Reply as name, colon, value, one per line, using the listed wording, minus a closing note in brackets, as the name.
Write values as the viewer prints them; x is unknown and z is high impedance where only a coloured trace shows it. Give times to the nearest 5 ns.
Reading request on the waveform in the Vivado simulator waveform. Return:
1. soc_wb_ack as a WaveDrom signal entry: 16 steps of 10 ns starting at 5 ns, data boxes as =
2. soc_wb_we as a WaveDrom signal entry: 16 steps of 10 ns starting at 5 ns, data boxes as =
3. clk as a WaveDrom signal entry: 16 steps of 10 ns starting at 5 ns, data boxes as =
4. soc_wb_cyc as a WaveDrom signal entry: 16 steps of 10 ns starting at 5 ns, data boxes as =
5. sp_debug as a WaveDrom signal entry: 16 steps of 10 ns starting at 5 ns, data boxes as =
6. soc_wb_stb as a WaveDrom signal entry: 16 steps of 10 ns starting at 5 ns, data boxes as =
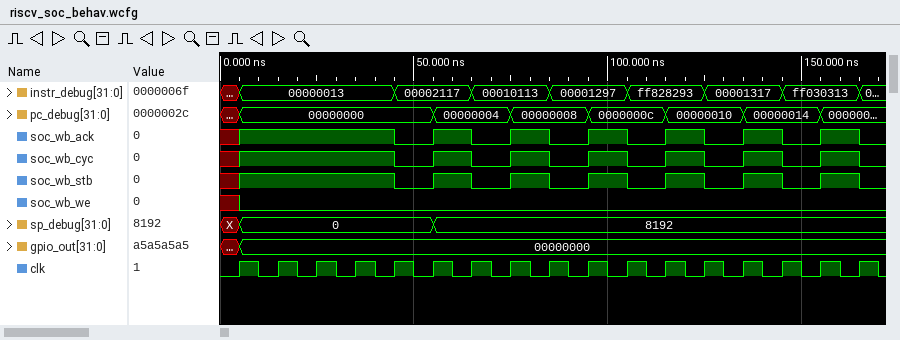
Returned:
soc_wb_ack as a WaveDrom signal entry: 16 steps of 10 ns starting at 5 ns, data boxes as =: {name: 'soc_wb_ack', wave: '1...010101010101'}
soc_wb_we as a WaveDrom signal entry: 16 steps of 10 ns starting at 5 ns, data boxes as =: {name: 'soc_wb_we', wave: '0...............'}
clk as a WaveDrom signal entry: 16 steps of 10 ns starting at 5 ns, data boxes as =: {name: 'clk', wave: 'p...............'}
soc_wb_cyc as a WaveDrom signal entry: 16 steps of 10 ns starting at 5 ns, data boxes as =: {name: 'soc_wb_cyc', wave: '1...010101010101'}
sp_debug as a WaveDrom signal entry: 16 steps of 10 ns starting at 5 ns, data boxes as =: {name: 'sp_debug', wave: '=....=..........', data: '0 8192'}
soc_wb_stb as a WaveDrom signal entry: 16 steps of 10 ns starting at 5 ns, data boxes as =: {name: 'soc_wb_stb', wave: '1...010101010101'}
